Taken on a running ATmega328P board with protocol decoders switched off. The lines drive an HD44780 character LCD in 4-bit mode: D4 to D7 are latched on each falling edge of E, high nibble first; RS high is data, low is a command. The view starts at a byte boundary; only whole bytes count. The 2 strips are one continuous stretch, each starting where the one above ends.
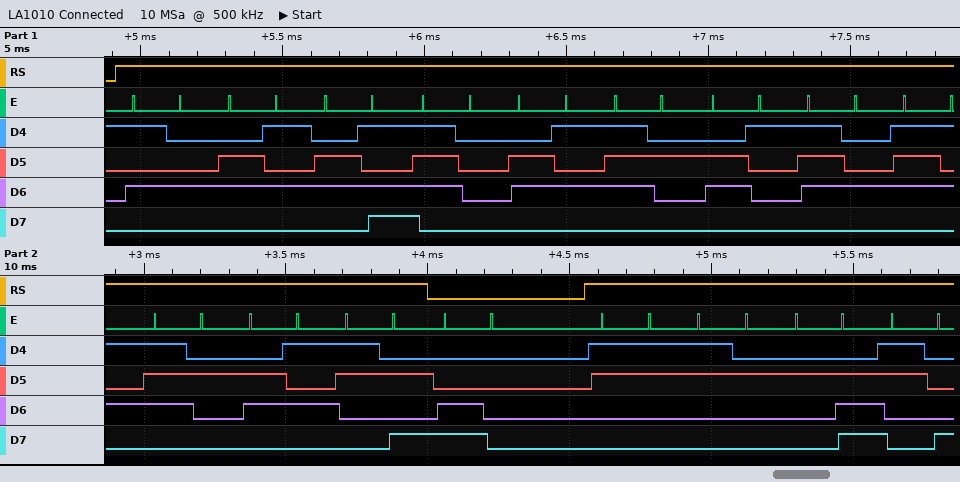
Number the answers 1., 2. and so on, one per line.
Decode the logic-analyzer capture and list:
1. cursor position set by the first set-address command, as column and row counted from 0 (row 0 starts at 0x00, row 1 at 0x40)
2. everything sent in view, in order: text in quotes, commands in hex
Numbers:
1. column 0, row 1
2. "Temperature:" 0xC0 "32.8"
